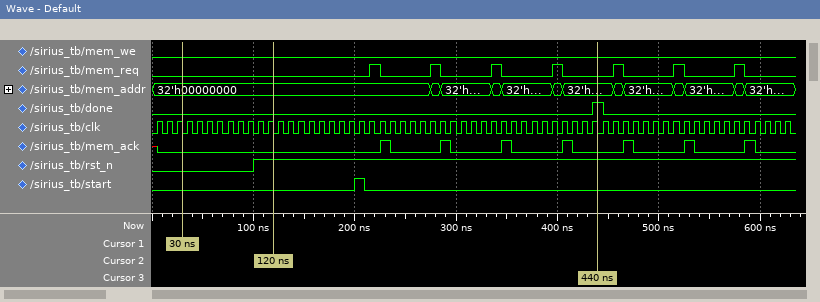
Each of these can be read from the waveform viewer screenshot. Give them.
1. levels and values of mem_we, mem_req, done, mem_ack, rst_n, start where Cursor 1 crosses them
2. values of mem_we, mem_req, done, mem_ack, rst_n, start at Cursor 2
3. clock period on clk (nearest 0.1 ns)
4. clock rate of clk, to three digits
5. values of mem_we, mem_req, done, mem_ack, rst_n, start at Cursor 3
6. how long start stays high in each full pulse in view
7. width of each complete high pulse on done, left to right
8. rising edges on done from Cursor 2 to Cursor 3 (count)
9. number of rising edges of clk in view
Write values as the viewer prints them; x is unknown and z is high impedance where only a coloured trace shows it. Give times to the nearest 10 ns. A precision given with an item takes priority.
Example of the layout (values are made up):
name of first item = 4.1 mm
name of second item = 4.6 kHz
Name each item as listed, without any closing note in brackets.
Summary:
levels and values of mem_we, mem_req, done, mem_ack, rst_n, start where Cursor 1 crosses them = mem_we=0, mem_req=0, done=0, mem_ack=0, rst_n=0, start=0
values of mem_we, mem_req, done, mem_ack, rst_n, start at Cursor 2 = mem_we=0, mem_req=0, done=0, mem_ack=0, rst_n=1, start=0
clock period on clk = 10 ns
clock rate of clk, to three digits = 100 MHz
values of mem_we, mem_req, done, mem_ack, rst_n, start at Cursor 3 = mem_we=0, mem_req=0, done=1, mem_ack=0, rst_n=1, start=0
how long start stays high in each full pulse in view = 10 ns
width of each complete high pulse on done, left to right = 10 ns
rising edges on done from Cursor 2 to Cursor 3 = 1
number of rising edges of clk in view = 63
